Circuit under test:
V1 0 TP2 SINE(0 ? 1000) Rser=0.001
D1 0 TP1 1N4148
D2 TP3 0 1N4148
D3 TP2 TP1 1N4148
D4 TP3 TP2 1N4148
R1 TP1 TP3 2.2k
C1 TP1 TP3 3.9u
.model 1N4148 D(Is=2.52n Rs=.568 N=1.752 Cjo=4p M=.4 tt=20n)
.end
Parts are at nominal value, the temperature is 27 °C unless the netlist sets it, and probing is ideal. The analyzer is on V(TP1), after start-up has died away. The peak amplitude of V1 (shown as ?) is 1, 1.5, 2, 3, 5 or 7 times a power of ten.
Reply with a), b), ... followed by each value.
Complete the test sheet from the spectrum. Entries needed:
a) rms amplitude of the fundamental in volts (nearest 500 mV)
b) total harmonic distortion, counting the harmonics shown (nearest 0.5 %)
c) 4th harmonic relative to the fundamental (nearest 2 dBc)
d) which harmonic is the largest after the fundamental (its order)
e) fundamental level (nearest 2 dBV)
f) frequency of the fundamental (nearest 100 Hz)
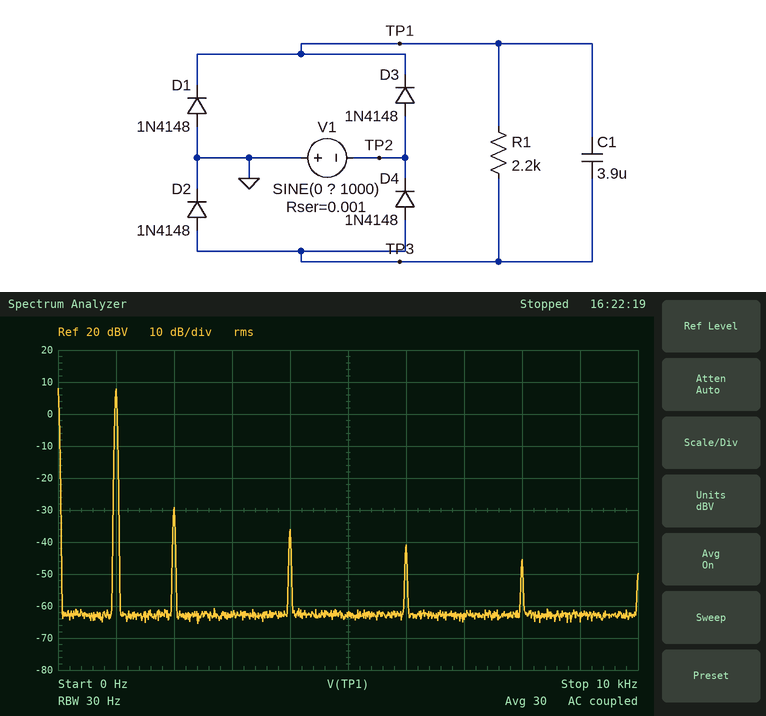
a) 2.5 V
b) 1.5 %
c) -44 dBc
d) 2
e) 8 dBV
f) 1.0 kHz
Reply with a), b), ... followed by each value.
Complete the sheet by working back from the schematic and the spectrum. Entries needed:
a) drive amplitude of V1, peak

a) 7 V
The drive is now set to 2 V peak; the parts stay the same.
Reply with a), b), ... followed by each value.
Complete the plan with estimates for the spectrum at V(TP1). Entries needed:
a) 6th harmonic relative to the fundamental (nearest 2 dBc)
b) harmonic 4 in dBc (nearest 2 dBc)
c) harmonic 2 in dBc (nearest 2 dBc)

a) -60 dBc
b) -52 dBc
c) -44 dBc
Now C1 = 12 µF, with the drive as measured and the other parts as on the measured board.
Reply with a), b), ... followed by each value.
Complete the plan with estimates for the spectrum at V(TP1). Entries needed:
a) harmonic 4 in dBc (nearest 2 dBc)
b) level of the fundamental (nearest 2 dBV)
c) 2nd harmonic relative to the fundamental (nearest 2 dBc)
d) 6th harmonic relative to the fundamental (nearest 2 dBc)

a) -54 dBc
b) 8 dBV
c) -46 dBc
d) -58 dBc
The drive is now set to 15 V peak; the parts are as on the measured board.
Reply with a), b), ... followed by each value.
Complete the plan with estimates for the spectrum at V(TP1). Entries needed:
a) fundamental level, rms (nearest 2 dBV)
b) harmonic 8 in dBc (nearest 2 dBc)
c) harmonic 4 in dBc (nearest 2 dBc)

a) 14 dBV
b) -50 dBc
c) -42 dBc
